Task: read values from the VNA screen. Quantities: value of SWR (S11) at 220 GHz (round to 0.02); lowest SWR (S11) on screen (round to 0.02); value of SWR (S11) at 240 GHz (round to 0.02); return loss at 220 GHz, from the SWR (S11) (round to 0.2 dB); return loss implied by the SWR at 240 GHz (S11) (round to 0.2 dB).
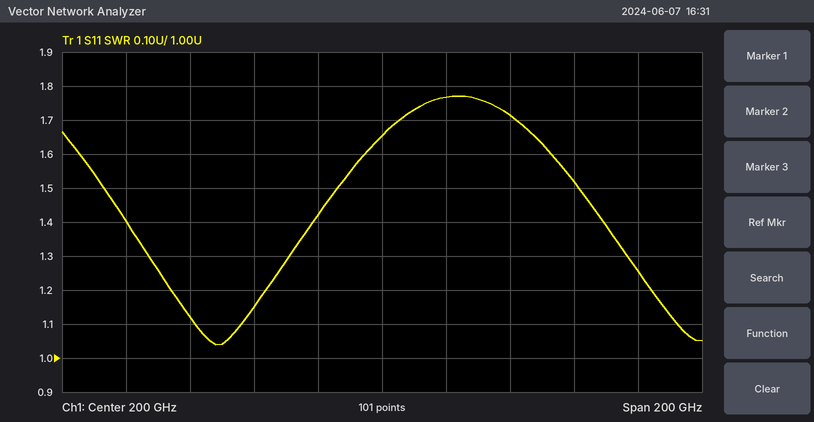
1.76
1.04
1.72
11.2 dB
11.6 dB
